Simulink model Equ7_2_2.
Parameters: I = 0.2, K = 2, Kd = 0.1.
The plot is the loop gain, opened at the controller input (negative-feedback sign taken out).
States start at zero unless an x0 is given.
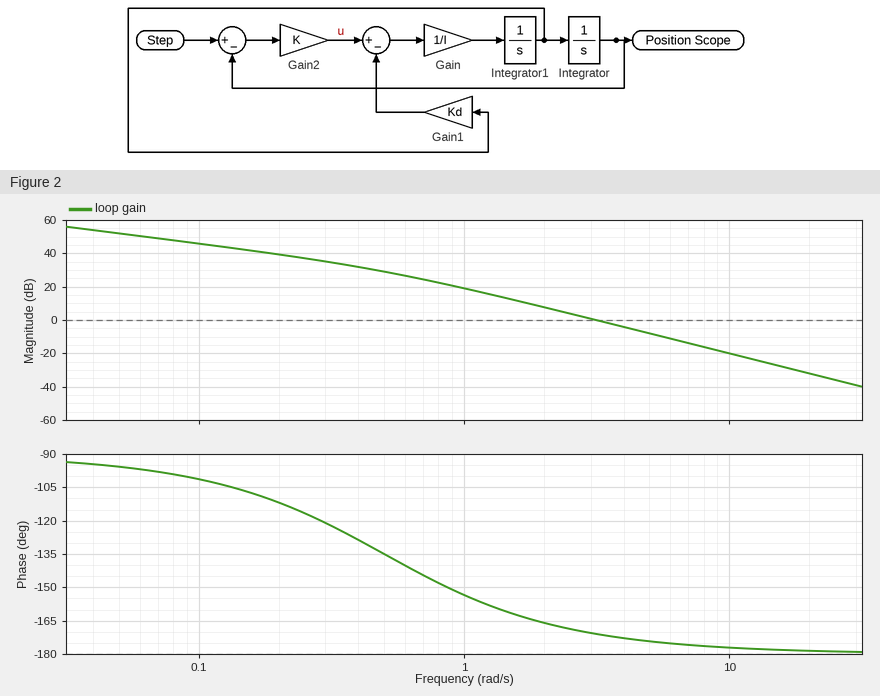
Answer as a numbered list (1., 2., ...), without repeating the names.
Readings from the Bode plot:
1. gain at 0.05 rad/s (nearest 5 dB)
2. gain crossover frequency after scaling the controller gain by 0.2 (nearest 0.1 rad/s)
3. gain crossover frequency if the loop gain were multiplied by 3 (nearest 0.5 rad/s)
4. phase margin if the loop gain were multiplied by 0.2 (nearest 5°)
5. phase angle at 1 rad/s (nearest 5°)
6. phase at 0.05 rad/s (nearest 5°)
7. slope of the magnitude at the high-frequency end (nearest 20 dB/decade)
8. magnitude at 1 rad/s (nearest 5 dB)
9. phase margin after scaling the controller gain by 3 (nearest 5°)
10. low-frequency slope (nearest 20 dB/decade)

1. 50 dB
2. 1.4 rad/s
3. 5.5 rad/s
4. 20°
5. -155°
6. -95°
7. -40 dB/decade
8. 20 dB
9. 5°
10. -20 dB/decade
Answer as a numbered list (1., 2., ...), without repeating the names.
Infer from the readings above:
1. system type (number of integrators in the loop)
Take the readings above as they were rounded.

1. 1
